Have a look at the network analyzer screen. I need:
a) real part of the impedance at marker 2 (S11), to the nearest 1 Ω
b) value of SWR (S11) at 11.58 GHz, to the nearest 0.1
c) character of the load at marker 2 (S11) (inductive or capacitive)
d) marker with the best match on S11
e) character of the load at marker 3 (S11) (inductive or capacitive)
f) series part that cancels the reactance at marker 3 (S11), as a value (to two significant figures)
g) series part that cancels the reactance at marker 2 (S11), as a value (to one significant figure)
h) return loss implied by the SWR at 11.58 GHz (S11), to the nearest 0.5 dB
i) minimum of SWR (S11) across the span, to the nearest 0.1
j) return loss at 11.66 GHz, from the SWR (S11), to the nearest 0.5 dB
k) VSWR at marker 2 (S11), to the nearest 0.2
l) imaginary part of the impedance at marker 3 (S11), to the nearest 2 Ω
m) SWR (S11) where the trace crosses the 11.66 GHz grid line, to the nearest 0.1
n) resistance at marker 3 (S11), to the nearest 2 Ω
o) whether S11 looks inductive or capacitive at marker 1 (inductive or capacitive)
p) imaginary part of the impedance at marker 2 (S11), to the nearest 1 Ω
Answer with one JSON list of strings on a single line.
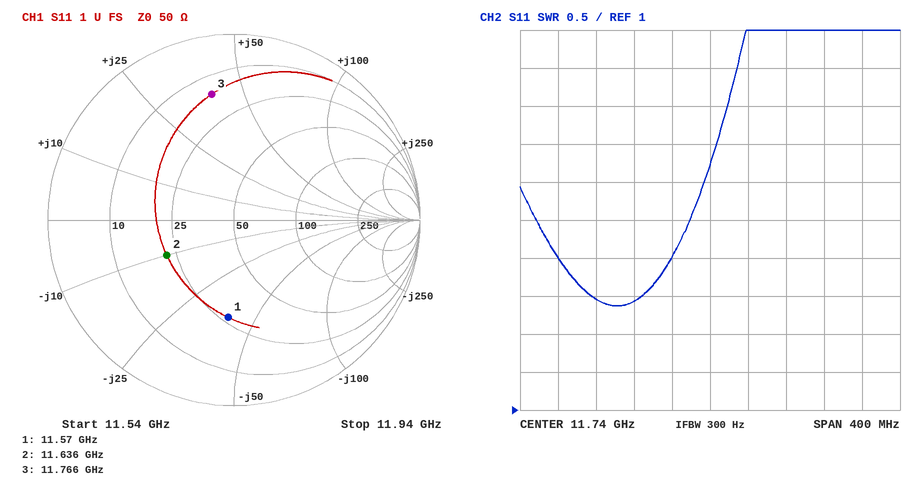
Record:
["22 Ω", "3.0", "capacitive", "marker 2", "inductive", "340 fF", "100 pH", "6.0 dB", "2.4", "7.5 dB", "2.4", "+40 Ω", "2.4", "16 Ω", "capacitive", "-10 Ω"]
